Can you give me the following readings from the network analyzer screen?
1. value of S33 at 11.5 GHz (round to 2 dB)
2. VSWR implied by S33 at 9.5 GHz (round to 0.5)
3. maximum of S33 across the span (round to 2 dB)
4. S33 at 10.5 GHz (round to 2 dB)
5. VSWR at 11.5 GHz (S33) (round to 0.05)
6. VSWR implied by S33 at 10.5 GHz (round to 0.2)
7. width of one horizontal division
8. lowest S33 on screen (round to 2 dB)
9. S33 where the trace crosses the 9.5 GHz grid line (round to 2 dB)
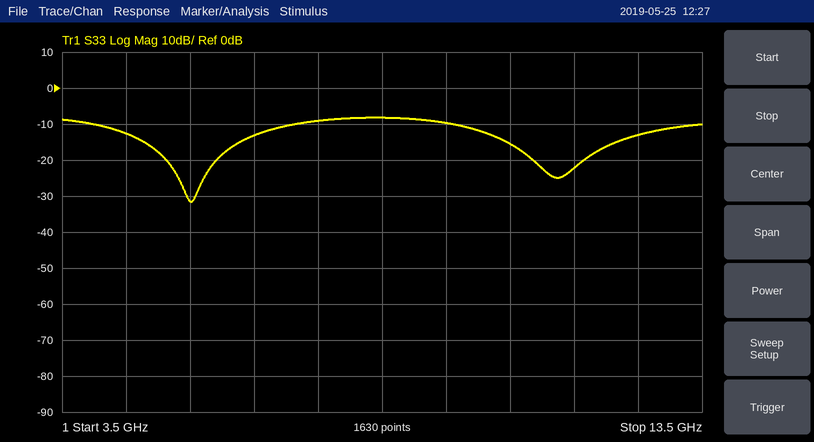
-22 dB
2.0
-8 dB
-16 dB
1.15
1.4
1 GHz
-32 dB
-10 dB
